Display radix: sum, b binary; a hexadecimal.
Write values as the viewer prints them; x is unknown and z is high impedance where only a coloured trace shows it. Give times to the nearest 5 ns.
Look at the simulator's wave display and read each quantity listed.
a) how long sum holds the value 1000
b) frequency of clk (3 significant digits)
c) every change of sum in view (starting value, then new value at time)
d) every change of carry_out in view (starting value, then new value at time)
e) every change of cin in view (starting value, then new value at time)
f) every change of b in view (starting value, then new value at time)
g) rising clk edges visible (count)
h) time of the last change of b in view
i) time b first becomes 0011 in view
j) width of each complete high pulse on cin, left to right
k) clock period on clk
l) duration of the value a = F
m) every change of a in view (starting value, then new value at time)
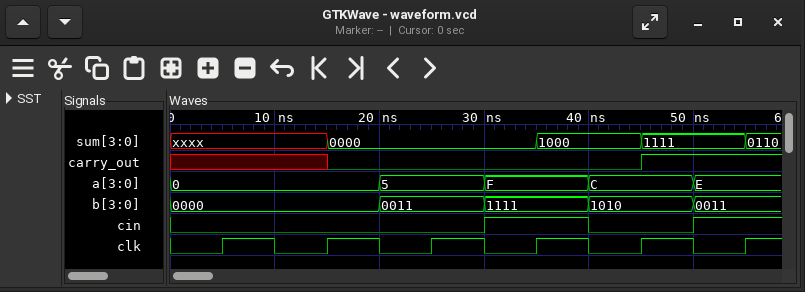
10 ns
100 MHz
xxxx, 0000 at 15 ns, 1000 at 35 ns, 1111 at 45 ns, 0110 at 55 ns
x, 0 at 15 ns, 1 at 45 ns
0, 1 at 30 ns, 0 at 40 ns, 1 at 50 ns
0000, 0011 at 20 ns, 1111 at 30 ns, 1010 at 40 ns, 0011 at 50 ns
6
50 ns
20 ns
10 ns
10 ns
10 ns
0, 5 at 20 ns, F at 30 ns, C at 40 ns, E at 50 ns
